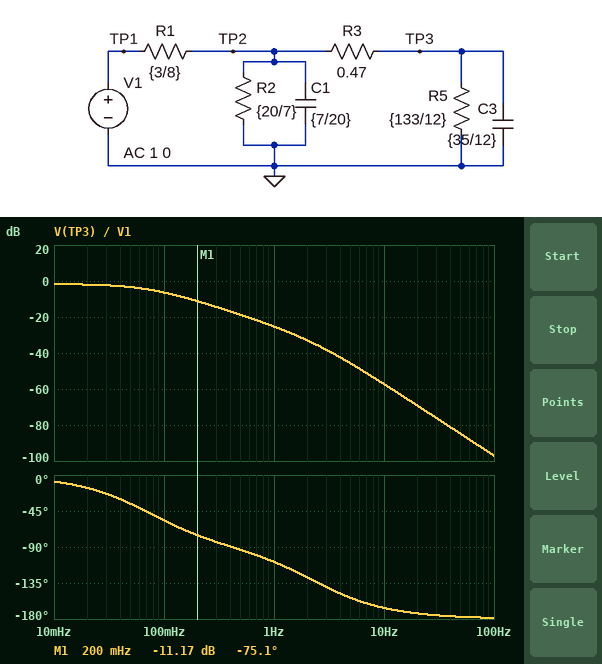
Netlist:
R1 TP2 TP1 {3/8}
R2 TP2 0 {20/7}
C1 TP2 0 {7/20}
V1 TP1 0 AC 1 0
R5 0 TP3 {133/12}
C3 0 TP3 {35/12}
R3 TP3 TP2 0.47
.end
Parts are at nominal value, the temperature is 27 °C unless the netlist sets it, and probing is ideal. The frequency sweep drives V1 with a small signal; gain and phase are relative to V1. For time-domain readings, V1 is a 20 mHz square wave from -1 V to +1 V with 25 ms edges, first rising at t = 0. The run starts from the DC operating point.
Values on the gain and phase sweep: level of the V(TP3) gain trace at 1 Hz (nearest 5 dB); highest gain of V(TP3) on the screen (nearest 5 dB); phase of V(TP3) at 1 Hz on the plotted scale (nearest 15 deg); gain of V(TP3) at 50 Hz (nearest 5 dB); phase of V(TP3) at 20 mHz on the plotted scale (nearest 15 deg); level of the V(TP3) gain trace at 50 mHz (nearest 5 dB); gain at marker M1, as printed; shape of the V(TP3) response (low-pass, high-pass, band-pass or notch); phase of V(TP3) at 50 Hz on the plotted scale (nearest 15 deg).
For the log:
-25 dB
0 dB
-105 deg
-85 dB
-15 deg
-5 dB
-11.17 dB
low-pass
-180 deg
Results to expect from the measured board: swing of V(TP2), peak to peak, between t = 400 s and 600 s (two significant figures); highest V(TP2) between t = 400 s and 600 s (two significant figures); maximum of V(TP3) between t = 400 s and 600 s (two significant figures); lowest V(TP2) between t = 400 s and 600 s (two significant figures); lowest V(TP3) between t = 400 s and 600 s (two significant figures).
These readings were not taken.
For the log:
1.7 V
860 mV
820 mV
-860 mV
-820 mV
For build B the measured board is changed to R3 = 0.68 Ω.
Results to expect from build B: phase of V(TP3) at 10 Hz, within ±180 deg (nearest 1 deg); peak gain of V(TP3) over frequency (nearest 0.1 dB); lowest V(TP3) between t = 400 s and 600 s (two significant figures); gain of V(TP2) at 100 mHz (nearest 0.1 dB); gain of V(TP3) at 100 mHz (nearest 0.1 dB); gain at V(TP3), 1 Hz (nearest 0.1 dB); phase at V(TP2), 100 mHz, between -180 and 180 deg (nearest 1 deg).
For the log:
-168 deg
-1.8 dB
-810 mV
-3.5 dB
-7.8 dB
-27.5 dB
-13 deg
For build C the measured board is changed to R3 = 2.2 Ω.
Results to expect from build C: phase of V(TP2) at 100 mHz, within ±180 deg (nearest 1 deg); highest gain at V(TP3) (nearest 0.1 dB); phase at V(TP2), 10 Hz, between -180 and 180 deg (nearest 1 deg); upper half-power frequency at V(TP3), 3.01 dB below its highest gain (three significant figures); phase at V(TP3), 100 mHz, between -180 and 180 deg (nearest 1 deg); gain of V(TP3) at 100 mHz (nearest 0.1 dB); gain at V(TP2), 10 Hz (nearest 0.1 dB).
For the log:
-5 deg
-2.9 dB
-81 deg
26.4 mHz
-79 deg
-14.7 dB
-18.4 dB
